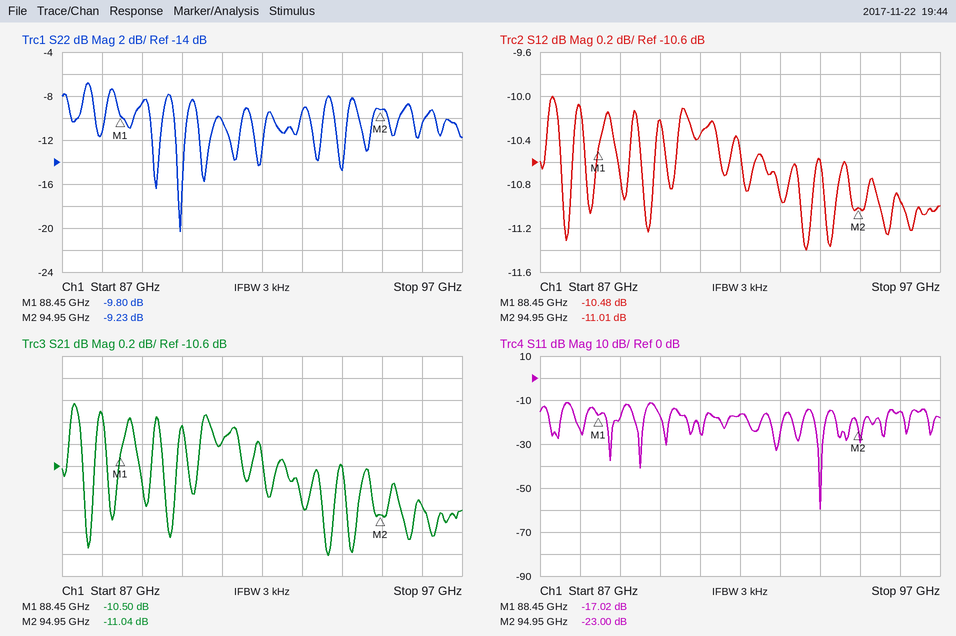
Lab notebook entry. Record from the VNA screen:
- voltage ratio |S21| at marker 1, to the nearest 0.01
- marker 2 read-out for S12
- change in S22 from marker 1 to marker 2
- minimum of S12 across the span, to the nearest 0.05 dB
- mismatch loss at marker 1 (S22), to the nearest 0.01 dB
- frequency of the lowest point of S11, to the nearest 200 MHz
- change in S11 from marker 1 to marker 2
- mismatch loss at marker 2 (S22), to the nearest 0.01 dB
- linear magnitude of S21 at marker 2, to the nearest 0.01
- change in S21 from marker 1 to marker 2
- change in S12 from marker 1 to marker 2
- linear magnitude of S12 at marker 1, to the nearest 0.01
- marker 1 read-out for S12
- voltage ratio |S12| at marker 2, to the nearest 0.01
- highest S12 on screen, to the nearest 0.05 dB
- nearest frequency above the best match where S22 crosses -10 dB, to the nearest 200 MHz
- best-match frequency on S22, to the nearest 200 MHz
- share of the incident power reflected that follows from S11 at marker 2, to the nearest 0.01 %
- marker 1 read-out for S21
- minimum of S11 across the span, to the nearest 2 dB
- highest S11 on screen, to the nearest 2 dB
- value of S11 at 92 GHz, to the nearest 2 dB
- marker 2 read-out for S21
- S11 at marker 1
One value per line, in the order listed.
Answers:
0.30
-11.01 dB
0.57 dB
-11.40 dB
0.48 dB
94.0 GHz
-5.98 dB
0.55 dB
0.28
-0.54 dB
-0.53 dB
0.30
-10.48 dB
0.28
-10.00 dB
90.2 GHz
90.0 GHz
0.50 %
-10.50 dB
-60 dB
-12 dB
-16 dB
-11.04 dB
-17.02 dB
